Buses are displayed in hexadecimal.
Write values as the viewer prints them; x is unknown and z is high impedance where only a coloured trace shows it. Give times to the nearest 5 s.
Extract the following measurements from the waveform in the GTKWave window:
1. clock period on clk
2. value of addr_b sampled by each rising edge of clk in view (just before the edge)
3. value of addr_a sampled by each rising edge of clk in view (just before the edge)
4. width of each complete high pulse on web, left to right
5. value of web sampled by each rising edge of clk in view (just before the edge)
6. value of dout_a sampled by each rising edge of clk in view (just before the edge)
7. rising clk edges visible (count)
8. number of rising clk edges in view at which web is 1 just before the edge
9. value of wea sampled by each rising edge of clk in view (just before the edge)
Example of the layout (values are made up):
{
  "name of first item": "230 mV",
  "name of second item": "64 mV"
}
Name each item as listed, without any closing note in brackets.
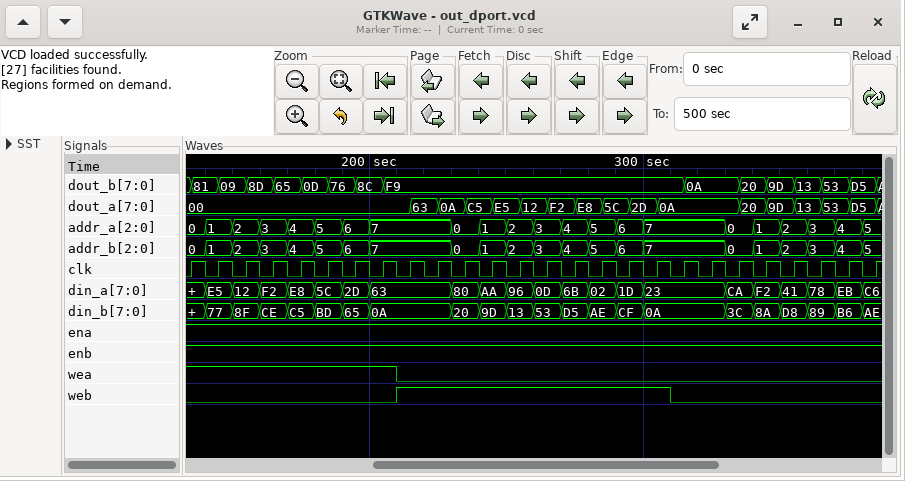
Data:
{
  "clock period on clk": "10 s",
  "value of addr_b sampled by each rising edge of clk in view": "0, 1, 2, 3, 4, 5, 6, 7, 7, 7, 0, 1, 2, 3, 4, 5, 6, 7, 7, 7, 0, 1, 2, 3, 4, 5",
  "value of addr_a sampled by each rising edge of clk in view": "0, 1, 2, 3, 4, 5, 6, 7, 7, 7, 0, 1, 2, 3, 4, 5, 6, 7, 7, 7, 0, 1, 2, 3, 4, 5",
  "width of each complete high pulse on web, left to right": "100 s",
  "value of web sampled by each rising edge of clk in view": "0 0 0 0 0 0 0 0 1 1 1 1 1 1 1 1 1 1 0 0 0 0 0 0 0 0",
  "value of dout_a sampled by each rising edge of clk in view": "00, 00, 00, 00, 00, 00, 00, 00, 00, 63, 0A, C5, E5, 12, F2, E8, 5C, 2D, 0A, 0A, 0A, 20, 9D, 13, 53, D5",
  "rising clk edges visible": "26",
  "number of rising clk edges in view at which web is 1 just before the edge": "10",
  "value of wea sampled by each rising edge of clk in view": "1 1 1 1 1 1 1 1 0 0 0 0 0 0 0 0 0 0 0 0 0 0 0 0 0 0"
}
